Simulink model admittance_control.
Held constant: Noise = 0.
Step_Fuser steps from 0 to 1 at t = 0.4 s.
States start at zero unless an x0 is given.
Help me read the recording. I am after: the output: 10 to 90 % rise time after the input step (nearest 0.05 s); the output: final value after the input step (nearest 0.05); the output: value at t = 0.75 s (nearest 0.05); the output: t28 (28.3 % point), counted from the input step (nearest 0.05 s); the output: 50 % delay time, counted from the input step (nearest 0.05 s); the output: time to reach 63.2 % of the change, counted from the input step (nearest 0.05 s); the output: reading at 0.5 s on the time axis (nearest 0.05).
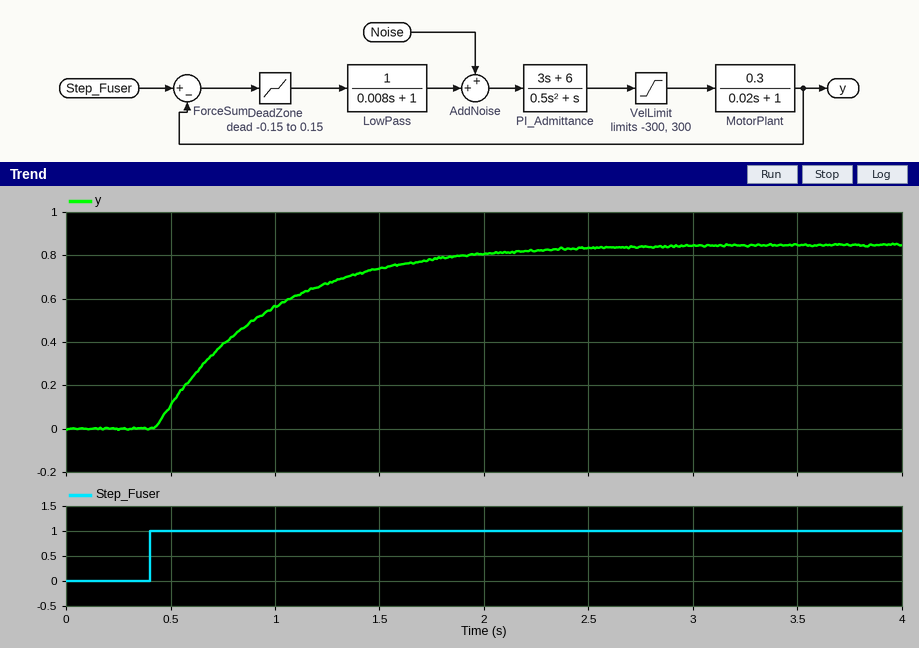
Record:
1.15 s
0.85
0.40
0.20 s
0.40 s
0.55 s
0.10
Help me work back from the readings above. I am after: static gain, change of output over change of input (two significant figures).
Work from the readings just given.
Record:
0.85
